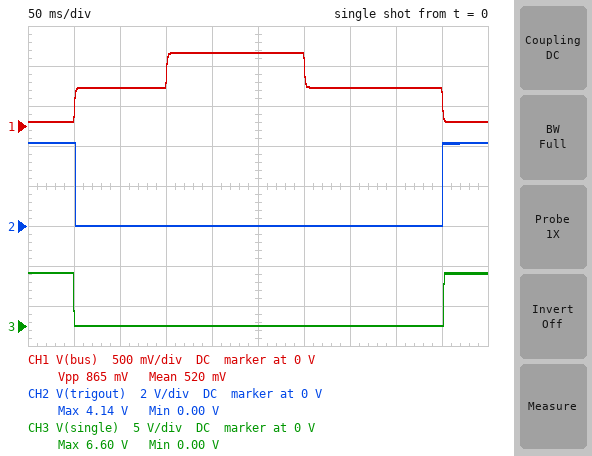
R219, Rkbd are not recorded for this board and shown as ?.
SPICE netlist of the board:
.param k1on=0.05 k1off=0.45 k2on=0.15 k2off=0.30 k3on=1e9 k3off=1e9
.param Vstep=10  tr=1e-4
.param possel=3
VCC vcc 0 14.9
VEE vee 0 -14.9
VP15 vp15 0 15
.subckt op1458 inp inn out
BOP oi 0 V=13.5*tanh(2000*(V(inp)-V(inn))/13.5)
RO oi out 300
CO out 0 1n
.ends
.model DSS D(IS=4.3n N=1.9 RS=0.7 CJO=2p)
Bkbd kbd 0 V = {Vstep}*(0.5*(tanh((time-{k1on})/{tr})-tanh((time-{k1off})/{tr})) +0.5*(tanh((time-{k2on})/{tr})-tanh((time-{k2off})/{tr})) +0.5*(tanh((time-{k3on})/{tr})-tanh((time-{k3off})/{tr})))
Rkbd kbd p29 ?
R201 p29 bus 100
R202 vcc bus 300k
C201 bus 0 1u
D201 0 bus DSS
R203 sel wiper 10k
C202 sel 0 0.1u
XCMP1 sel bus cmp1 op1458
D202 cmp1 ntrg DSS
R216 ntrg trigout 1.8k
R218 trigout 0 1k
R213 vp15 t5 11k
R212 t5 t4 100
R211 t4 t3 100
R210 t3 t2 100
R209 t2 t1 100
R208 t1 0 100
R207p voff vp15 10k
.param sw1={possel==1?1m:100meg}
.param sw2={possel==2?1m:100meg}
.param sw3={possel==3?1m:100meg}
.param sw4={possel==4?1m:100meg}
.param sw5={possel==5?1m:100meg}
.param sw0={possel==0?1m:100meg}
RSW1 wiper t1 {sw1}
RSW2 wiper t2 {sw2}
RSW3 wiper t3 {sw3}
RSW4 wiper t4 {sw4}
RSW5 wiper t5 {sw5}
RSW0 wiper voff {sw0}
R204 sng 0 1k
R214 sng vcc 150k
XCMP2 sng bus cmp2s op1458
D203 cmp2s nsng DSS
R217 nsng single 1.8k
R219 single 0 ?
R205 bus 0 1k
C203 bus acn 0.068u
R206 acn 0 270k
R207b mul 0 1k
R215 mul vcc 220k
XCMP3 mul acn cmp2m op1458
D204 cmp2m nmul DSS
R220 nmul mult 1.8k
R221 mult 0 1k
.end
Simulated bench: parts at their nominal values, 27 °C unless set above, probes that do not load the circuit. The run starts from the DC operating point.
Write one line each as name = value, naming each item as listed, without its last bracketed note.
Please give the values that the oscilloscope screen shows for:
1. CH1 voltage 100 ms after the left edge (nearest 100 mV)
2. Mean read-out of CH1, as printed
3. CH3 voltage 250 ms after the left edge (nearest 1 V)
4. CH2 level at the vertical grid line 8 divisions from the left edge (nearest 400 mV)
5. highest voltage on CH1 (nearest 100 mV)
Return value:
CH1 voltage 100 ms after the left edge = 500 mV
Mean read-out of CH1, as printed = 520 mV
CH3 voltage 250 ms after the left edge = 0 V
CH2 level at the vertical grid line 8 divisions from the left edge = 0 V
highest voltage on CH1 = 900 mV
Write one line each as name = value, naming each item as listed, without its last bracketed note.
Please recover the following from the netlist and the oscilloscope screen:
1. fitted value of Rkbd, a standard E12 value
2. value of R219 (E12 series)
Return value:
fitted value of Rkbd, a standard E12 value = 22 kΩ
value of R219 = 2.2 kΩ
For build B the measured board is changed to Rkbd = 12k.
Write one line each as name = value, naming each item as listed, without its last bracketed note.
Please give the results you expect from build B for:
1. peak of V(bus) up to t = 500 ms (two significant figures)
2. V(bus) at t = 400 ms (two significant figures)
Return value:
peak of V(bus) up to t = 500 ms = 1.6 V
V(bus) at t = 400 ms = 810 mV
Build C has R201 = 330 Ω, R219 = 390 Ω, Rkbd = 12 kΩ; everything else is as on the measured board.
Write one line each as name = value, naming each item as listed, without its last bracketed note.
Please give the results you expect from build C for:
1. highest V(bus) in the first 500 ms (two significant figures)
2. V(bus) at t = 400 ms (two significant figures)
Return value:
highest V(bus) in the first 500 ms = 1.5 V
V(bus) at t = 400 ms = 790 mV
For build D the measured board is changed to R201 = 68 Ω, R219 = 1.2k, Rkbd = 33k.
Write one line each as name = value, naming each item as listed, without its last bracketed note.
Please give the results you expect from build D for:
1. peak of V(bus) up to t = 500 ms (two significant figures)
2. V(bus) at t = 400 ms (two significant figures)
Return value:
peak of V(bus) up to t = 500 ms = 630 mV
V(bus) at t = 400 ms = 340 mV
